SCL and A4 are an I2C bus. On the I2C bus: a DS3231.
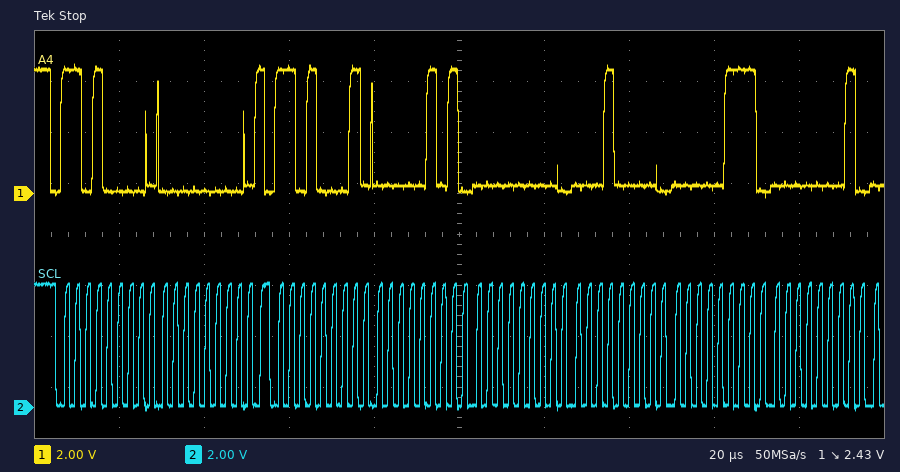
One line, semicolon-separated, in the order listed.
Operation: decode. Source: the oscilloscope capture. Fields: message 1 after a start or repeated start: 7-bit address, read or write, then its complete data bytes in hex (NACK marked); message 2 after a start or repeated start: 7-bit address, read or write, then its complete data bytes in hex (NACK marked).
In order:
0x68 write: 00; 0x68 read: 05 00 10 07 01
